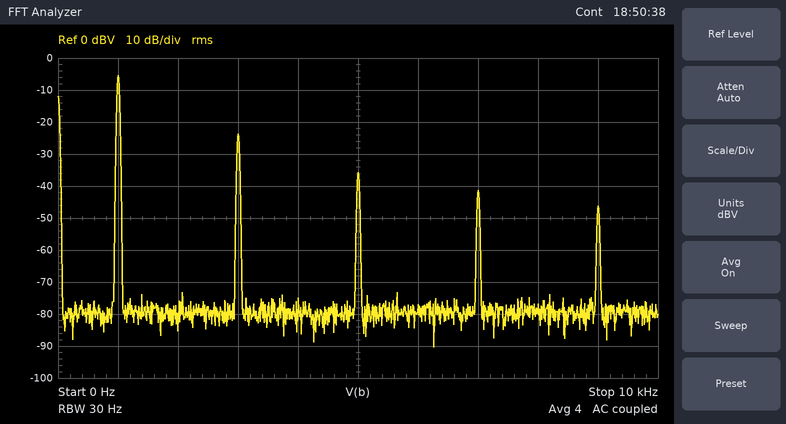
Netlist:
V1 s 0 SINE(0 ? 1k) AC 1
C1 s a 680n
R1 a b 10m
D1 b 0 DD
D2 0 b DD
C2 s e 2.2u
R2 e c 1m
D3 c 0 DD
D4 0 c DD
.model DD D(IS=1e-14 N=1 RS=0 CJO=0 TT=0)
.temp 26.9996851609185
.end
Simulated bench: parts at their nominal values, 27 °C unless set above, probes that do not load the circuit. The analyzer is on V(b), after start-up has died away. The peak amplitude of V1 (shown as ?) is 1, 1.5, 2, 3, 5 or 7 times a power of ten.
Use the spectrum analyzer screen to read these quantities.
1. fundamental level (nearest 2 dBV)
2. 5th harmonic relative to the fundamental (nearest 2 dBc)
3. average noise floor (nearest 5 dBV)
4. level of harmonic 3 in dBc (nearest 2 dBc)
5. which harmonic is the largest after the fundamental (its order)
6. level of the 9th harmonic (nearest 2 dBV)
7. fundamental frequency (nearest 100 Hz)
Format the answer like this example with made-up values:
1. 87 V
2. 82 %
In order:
1. -6 dBV
2. -30 dBc
3. -80 dBV
4. -18 dBc
5. 3
6. -46 dBV
7. 1.0 kHz
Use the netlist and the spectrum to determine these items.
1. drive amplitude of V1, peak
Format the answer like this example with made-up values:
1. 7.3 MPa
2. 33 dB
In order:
1. 1 V
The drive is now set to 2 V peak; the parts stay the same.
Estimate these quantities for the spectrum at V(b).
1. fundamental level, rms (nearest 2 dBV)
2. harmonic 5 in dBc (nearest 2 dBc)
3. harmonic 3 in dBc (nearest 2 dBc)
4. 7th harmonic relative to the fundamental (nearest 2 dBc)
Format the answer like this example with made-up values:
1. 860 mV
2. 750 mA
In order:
1. -4 dBV
2. -24 dBc
3. -14 dBc
4. -32 dBc
